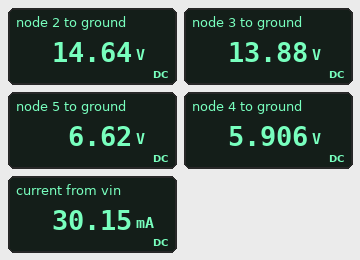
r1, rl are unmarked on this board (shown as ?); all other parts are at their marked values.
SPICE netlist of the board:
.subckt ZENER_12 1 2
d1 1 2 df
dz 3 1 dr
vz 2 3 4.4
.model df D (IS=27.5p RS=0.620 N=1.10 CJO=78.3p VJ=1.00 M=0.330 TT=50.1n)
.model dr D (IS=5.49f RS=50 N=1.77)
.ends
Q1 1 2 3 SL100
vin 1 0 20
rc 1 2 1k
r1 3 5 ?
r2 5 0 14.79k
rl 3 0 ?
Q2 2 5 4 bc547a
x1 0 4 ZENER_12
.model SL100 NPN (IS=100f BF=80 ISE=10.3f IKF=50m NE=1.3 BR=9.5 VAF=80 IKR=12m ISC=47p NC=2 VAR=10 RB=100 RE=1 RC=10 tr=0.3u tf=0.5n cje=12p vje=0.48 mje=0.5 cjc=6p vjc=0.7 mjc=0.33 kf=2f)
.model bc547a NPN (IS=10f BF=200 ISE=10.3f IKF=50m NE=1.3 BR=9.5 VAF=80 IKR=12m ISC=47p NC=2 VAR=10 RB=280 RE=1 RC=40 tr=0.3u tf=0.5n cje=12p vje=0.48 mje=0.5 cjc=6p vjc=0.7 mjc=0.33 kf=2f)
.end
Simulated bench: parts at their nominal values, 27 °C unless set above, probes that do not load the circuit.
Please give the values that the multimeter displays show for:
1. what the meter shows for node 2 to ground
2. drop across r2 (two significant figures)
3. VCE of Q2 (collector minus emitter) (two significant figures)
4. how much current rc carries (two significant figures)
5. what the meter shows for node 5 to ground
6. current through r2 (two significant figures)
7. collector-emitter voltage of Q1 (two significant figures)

14.64 V
6.6 V
8.7 V
5.4 mA
6.62 V
450 µA
6.1 V
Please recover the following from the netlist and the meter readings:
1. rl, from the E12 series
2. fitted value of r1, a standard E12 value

560 Ω
15 kΩ
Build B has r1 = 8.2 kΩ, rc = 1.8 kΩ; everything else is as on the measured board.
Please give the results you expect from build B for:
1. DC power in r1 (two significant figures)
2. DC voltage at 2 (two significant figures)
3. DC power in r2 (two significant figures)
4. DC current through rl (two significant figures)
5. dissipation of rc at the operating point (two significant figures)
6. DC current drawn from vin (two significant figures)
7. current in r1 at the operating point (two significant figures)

1.9 mW
11 V
2.9 mW
19 mA
42 mW
24 mA
480 µA
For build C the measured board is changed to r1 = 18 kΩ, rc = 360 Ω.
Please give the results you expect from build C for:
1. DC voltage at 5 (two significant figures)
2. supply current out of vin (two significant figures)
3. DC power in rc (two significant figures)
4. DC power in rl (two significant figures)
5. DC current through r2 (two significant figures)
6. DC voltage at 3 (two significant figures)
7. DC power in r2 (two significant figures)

6.8 V
37 mA
26 mW
470 mW
460 µA
16 V
3.1 mW
